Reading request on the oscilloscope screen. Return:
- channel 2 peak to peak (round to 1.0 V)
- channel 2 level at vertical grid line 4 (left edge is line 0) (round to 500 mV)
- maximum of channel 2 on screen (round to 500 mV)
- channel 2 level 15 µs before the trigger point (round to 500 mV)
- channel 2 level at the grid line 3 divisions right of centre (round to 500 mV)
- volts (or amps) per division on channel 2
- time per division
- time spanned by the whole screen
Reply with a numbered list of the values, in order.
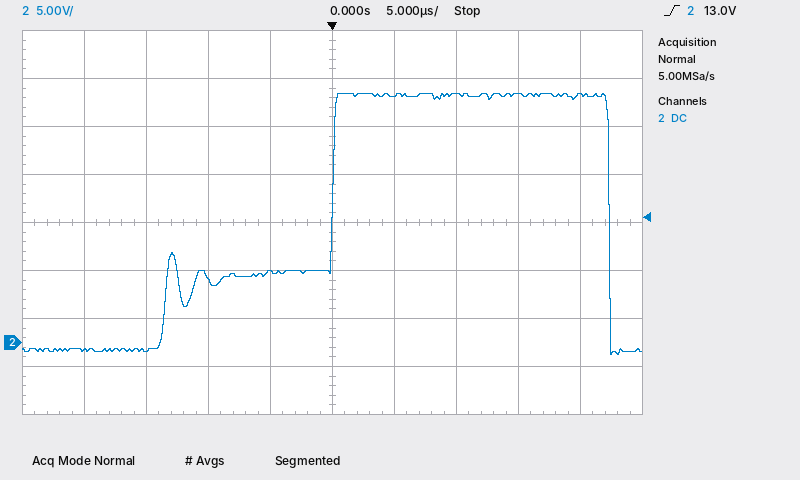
1. 27.0 V
2. 7.5 V
3. 26.0 V
4. -1.0 V
5. 26.0 V
6. 5 V
7. 5 µs
8. 50 µs
